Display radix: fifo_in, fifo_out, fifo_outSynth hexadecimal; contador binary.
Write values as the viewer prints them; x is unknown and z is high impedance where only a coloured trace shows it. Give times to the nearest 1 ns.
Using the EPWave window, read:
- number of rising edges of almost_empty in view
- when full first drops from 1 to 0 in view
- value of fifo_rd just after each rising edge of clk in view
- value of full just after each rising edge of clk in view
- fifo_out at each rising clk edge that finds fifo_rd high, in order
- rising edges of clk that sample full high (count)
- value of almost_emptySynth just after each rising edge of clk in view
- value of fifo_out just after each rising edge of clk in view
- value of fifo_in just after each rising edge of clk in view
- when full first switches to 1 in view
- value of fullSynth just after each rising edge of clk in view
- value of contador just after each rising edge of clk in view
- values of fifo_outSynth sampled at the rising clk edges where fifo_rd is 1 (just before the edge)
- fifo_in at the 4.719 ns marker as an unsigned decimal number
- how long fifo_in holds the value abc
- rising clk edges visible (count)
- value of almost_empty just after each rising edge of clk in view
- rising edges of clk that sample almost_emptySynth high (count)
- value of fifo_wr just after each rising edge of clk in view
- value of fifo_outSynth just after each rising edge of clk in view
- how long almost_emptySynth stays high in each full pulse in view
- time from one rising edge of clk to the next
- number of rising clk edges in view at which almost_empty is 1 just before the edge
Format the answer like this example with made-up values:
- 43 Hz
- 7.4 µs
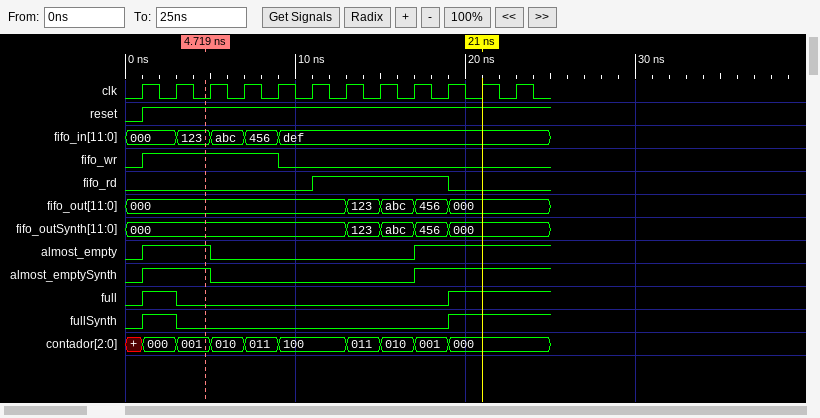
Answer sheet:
- 2
- 3 ns
- 0 0 0 0 0 1 1 1 1 0 0 0
- 1 0 0 0 0 0 0 0 0 1 1 1
- 000, 123, abc, 456
- 3
- 1 1 0 0 0 0 0 0 1 1 1 1
- 000, 000, 000, 000, 000, 000, 123, abc, 456, 000, 000, 000
- 000, 123, abc, 456, def, def, def, def, def, def, def, def
- 1 ns
- 1 0 0 0 0 0 0 0 0 1 1 1
- 000, 001, 010, 011, 100, 100, 011, 010, 001, 000, 000, 000
- 000, 123, abc, 456
- 291
- 2 ns
- 12
- 1 1 0 0 0 0 0 0 1 1 1 1
- 5
- 1 1 1 1 0 0 0 0 0 0 0 0
- 000, 000, 000, 000, 000, 000, 123, abc, 456, 000, 000, 000
- 4 ns
- 2 ns
- 5
